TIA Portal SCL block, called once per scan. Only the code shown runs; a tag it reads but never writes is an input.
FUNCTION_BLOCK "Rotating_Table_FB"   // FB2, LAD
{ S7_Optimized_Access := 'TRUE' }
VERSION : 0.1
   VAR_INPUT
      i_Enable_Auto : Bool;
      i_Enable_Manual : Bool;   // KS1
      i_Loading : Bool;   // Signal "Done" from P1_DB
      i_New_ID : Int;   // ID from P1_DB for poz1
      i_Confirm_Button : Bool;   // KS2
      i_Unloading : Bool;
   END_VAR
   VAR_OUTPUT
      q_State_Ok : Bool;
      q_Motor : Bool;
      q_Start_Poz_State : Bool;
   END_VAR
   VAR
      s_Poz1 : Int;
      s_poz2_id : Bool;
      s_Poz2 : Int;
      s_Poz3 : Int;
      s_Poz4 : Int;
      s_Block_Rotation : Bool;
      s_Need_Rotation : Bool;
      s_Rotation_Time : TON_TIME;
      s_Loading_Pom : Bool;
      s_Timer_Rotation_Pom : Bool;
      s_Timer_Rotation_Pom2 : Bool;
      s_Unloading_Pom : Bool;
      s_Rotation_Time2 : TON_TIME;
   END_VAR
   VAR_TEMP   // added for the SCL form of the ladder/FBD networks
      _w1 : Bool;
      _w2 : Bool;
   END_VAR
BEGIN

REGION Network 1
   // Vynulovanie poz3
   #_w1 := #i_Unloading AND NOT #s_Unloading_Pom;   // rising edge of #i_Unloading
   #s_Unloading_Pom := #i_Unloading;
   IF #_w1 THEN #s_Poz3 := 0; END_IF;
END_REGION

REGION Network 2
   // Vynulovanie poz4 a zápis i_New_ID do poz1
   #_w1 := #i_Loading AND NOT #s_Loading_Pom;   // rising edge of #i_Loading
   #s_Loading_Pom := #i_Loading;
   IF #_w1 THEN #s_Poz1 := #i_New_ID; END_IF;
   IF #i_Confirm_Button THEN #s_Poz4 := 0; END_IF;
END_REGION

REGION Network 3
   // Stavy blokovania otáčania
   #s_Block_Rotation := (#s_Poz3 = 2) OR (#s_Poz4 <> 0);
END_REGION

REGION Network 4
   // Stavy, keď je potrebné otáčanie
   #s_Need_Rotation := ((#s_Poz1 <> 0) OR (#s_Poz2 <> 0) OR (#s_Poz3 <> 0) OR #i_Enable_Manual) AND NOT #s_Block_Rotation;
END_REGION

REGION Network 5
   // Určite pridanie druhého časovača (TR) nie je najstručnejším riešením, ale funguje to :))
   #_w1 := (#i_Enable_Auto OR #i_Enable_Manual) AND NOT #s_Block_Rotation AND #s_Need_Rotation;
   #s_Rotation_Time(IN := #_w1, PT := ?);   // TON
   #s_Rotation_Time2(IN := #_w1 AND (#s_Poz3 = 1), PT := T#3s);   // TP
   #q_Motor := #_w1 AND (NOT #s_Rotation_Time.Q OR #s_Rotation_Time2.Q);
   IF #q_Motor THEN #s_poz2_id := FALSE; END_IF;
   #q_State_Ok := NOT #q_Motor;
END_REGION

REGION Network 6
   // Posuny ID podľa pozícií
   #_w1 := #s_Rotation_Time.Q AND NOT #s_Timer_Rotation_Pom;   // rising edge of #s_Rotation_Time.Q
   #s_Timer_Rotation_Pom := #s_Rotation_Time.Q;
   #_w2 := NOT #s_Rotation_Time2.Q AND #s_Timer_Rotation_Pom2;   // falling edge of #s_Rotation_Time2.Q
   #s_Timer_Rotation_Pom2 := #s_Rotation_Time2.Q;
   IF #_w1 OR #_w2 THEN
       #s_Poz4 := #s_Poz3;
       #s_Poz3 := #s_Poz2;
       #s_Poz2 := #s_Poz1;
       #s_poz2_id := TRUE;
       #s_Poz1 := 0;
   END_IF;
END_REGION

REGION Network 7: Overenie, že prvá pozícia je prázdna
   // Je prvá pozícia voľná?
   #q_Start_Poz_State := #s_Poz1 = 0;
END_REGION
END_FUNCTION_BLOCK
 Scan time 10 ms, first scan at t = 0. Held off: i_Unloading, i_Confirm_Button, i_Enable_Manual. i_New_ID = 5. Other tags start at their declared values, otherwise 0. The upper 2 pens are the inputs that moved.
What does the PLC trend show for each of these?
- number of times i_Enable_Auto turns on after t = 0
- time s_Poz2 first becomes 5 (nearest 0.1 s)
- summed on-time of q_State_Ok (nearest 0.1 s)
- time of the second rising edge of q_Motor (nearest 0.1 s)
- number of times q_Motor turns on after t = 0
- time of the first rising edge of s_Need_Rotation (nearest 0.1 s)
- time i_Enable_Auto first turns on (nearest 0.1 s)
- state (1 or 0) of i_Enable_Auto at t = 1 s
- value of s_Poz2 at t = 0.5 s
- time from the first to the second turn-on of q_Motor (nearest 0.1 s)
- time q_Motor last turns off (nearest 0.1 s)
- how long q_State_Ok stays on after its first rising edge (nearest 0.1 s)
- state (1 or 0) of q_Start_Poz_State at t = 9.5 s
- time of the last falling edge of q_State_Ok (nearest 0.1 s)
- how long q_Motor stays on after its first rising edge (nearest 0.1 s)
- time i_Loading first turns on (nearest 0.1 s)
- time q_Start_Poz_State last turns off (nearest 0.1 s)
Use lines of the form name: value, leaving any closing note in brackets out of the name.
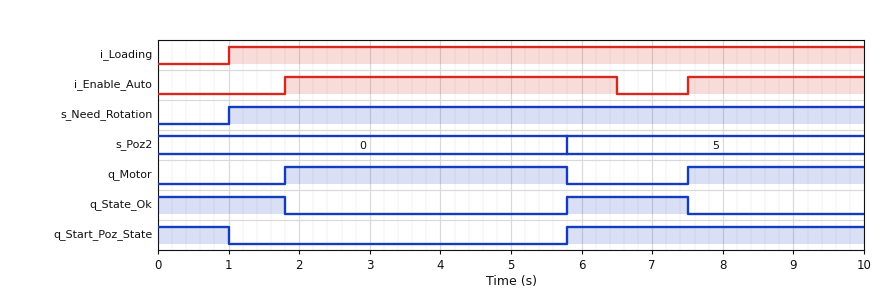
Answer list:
number of times i_Enable_Auto turns on after t = 0: 2
time s_Poz2 first becomes 5: 5.8 s
summed on-time of q_State_Ok: 3.5 s
time of the second rising edge of q_Motor: 7.5 s
number of times q_Motor turns on after t = 0: 2
time of the first rising edge of s_Need_Rotation: 1.0 s
time i_Enable_Auto first turns on: 1.8 s
state (1 or 0) of i_Enable_Auto at t = 1 s: 0
value of s_Poz2 at t = 0.5 s: 0
time from the first to the second turn-on of q_Motor: 5.7 s
time q_Motor last turns off: 5.8 s
how long q_State_Ok stays on after its first rising edge: 1.7 s
state (1 or 0) of q_Start_Poz_State at t = 9.5 s: 1
time of the last falling edge of q_State_Ok: 7.5 s
how long q_Motor stays on after its first rising edge: 4.0 s
time i_Loading first turns on: 1.0 s
time q_Start_Poz_State last turns off: 1.0 s
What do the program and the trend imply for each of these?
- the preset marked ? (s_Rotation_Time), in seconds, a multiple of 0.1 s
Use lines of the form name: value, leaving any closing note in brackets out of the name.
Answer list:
the preset marked ? (s_Rotation_Time), in seconds, a multiple of 0.1 s: 4.0 s
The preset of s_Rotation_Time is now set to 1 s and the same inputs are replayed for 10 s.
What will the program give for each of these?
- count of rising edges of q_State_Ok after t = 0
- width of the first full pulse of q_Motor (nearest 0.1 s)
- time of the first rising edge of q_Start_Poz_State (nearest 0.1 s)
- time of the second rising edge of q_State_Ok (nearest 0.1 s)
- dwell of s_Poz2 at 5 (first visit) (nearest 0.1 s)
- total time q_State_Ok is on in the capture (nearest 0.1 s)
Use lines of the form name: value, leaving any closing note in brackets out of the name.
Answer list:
count of rising edges of q_State_Ok after t = 0: 2
width of the first full pulse of q_Motor: 1.0 s
time of the first rising edge of q_Start_Poz_State: 2.8 s
time of the second rising edge of q_State_Ok: 8.5 s
dwell of s_Poz2 at 5 (first visit): 5.7 s
total time q_State_Ok is on in the capture: 8.0 s
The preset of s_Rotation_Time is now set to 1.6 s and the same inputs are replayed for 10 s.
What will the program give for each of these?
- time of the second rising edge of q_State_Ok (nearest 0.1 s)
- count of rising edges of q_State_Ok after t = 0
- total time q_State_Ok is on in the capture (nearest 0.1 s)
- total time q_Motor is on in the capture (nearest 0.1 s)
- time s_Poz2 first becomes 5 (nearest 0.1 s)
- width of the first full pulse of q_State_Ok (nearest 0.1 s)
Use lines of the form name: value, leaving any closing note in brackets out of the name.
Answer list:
time of the second rising edge of q_State_Ok: 9.1 s
count of rising edges of q_State_Ok after t = 0: 2
total time q_State_Ok is on in the capture: 6.8 s
total time q_Motor is on in the capture: 3.2 s
time s_Poz2 first becomes 5: 3.4 s
width of the first full pulse of q_State_Ok: 4.1 s
